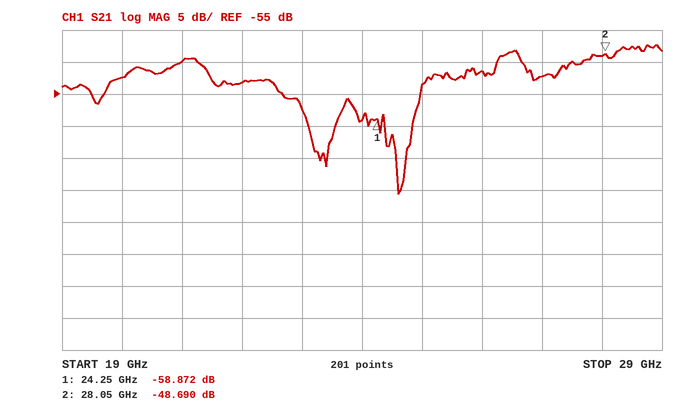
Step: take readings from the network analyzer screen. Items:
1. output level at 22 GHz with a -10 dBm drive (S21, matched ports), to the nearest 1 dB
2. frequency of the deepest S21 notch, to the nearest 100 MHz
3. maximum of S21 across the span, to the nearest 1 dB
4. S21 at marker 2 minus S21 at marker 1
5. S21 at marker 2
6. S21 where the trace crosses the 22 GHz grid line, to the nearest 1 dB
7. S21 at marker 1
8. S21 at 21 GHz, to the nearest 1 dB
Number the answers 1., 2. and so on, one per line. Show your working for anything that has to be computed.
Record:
1. -10 dBm + (-53 dB) = -63 dBm
2. 24.6 GHz
3. -47 dB
4. -48.69 − (-58.872) = 10.182 dB
5. -48.690 dB
6. -53 dB
7. -58.872 dB
8. -50 dB
